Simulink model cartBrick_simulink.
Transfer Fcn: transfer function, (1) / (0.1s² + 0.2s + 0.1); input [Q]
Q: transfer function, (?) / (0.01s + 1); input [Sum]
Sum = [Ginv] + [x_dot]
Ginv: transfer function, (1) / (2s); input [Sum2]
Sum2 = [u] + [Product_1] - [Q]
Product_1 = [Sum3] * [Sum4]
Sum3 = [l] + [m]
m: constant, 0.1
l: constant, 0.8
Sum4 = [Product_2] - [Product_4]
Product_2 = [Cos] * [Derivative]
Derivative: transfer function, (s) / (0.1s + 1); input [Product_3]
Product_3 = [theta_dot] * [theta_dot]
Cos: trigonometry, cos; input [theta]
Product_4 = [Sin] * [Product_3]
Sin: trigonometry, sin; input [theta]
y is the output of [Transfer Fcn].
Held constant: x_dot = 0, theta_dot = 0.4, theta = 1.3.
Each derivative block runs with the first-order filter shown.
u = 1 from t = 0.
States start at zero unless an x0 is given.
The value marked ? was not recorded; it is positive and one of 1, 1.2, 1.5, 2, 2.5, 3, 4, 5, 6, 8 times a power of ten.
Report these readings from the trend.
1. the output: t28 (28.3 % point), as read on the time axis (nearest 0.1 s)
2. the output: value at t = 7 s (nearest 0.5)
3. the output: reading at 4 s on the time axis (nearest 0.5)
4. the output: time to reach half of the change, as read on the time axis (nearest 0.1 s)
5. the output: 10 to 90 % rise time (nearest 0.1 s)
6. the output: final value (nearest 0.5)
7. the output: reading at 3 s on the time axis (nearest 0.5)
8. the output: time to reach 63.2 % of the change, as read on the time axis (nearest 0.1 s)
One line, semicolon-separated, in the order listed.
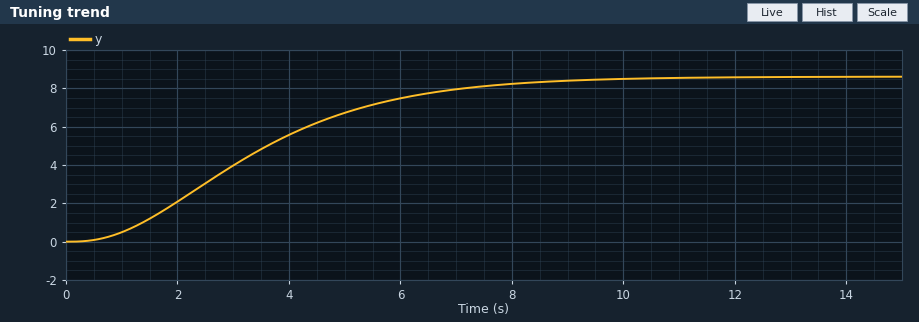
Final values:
2.2 s; 8.0; 5.5; 3.2 s; 5.2 s; 8.5; 4.0; 3.9 s
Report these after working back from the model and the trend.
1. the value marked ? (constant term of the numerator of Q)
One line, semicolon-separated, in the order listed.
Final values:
1.2
